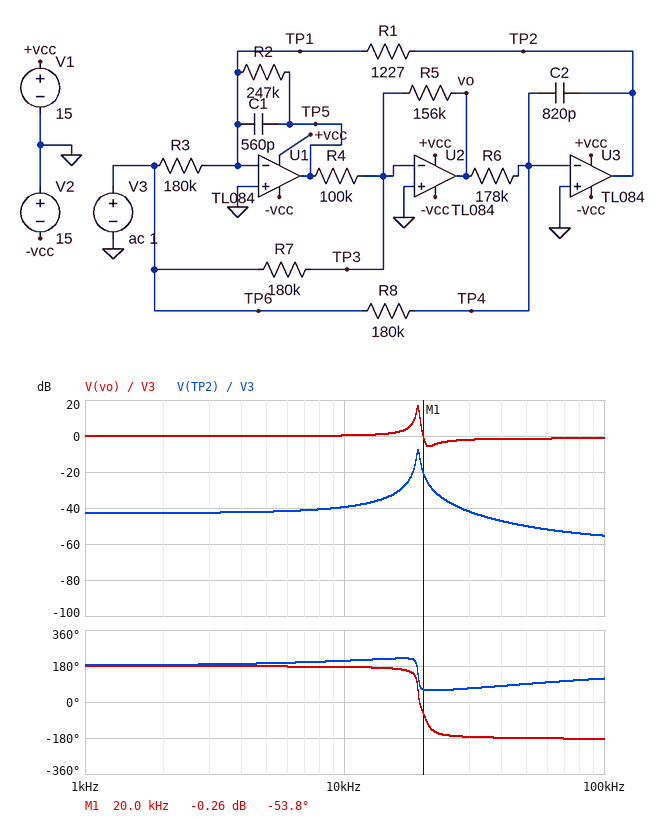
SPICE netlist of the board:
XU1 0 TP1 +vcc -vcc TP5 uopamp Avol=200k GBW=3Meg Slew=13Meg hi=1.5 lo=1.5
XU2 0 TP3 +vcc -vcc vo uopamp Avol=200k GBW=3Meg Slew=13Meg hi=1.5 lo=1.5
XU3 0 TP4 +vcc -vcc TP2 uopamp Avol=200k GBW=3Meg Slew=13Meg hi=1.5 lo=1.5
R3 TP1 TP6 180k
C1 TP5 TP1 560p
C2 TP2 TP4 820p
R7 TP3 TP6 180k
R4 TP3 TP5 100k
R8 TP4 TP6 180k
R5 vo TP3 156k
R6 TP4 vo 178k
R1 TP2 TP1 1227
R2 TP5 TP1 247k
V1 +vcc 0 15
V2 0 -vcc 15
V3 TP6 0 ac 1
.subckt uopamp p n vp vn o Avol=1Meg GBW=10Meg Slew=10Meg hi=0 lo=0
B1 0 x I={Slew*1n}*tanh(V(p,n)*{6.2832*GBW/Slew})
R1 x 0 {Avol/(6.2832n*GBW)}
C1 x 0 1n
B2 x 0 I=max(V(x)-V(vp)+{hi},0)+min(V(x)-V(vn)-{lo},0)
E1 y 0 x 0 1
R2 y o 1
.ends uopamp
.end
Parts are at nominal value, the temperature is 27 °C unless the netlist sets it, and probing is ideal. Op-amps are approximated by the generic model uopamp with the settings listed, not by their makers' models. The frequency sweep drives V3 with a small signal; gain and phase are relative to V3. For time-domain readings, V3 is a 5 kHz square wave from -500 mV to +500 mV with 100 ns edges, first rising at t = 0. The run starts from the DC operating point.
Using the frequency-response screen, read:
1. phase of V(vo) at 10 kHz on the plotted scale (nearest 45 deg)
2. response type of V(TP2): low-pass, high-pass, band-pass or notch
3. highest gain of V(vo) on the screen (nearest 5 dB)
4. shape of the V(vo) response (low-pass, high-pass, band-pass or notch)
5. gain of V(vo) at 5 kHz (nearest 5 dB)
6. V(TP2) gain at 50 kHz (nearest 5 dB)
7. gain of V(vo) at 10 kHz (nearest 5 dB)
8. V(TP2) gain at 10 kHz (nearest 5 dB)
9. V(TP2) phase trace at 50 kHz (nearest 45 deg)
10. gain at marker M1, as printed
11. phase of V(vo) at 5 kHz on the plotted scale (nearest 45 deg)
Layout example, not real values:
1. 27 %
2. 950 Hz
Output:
1. 180 deg
2. low-pass
3. 15 dB
4. band-pass
5. 0 dB
6. -50 dB
7. 0 dB
8. -40 dB
9. 90 deg
10. -0.26 dB
11. 180 deg
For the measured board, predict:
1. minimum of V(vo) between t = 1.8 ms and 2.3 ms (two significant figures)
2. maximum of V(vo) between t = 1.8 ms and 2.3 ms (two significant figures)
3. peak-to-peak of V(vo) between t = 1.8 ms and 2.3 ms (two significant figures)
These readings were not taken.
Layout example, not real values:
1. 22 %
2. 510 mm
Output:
1. -580 mV
2. 580 mV
3. 1.2 V
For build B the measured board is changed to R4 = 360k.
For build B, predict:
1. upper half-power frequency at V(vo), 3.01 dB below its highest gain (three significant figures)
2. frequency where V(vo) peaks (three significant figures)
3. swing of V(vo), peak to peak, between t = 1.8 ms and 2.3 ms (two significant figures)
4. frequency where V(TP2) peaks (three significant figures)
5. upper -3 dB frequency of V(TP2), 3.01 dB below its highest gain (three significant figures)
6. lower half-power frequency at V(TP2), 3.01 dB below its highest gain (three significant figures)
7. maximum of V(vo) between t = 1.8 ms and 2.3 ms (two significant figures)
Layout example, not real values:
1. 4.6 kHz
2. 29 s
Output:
1. 10.2 kHz
2. 9.76 kHz
3. 1.1 V
4. 10.1 kHz
5. 10.5 kHz
6. 9.61 kHz
7. 560 mV
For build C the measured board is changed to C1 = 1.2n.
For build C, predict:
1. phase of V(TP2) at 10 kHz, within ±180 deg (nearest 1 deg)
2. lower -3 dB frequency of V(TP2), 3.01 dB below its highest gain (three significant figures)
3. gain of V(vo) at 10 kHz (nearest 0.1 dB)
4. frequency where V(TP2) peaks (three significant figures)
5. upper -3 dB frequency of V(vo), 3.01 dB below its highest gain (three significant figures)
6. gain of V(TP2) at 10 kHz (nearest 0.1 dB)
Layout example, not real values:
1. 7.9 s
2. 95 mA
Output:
1. -133 deg
2. 13.2 kHz
3. 1.2 dB
4. 13.3 kHz
5. 13.4 kHz
6. -32.8 dB
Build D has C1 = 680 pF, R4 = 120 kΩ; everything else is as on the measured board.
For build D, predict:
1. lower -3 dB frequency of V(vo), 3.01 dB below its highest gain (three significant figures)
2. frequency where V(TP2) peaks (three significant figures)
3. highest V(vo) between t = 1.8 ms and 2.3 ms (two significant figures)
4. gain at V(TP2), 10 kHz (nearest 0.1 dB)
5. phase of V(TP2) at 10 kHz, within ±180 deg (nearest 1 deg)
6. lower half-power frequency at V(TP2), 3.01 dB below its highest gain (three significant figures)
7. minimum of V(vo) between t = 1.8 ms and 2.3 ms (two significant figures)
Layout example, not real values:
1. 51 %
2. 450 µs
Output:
1. 15.6 kHz
2. 15.9 kHz
3. 750 mV
4. -36.9 dB
5. -145 deg
6. 15.7 kHz
7. -760 mV
